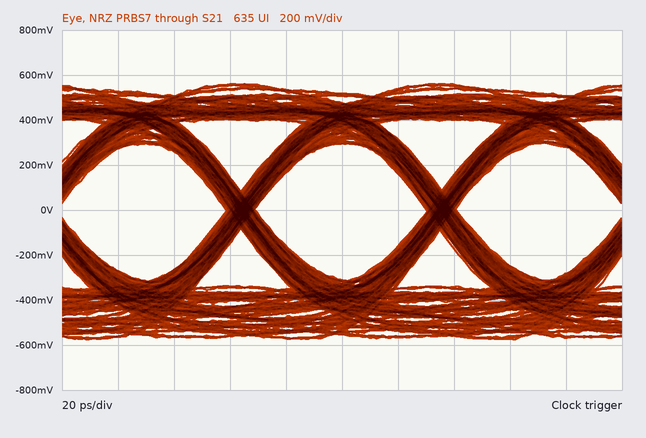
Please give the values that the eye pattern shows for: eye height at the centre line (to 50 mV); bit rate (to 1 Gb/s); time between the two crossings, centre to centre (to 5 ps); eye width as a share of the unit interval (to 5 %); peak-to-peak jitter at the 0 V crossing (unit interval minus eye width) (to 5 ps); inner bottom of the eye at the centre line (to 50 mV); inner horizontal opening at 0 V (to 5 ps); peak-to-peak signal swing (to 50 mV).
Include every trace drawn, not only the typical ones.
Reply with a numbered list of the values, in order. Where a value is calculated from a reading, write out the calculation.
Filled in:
1. 600 mV
2. 14 Gb/s
3. 70 ps
4. 60 ps / 70 ps ≈ 85.7 %, so 85 % to the nearest 5 %
5. 10 ps
6. -300 mV
7. 60 ps
8. 1.15 V
